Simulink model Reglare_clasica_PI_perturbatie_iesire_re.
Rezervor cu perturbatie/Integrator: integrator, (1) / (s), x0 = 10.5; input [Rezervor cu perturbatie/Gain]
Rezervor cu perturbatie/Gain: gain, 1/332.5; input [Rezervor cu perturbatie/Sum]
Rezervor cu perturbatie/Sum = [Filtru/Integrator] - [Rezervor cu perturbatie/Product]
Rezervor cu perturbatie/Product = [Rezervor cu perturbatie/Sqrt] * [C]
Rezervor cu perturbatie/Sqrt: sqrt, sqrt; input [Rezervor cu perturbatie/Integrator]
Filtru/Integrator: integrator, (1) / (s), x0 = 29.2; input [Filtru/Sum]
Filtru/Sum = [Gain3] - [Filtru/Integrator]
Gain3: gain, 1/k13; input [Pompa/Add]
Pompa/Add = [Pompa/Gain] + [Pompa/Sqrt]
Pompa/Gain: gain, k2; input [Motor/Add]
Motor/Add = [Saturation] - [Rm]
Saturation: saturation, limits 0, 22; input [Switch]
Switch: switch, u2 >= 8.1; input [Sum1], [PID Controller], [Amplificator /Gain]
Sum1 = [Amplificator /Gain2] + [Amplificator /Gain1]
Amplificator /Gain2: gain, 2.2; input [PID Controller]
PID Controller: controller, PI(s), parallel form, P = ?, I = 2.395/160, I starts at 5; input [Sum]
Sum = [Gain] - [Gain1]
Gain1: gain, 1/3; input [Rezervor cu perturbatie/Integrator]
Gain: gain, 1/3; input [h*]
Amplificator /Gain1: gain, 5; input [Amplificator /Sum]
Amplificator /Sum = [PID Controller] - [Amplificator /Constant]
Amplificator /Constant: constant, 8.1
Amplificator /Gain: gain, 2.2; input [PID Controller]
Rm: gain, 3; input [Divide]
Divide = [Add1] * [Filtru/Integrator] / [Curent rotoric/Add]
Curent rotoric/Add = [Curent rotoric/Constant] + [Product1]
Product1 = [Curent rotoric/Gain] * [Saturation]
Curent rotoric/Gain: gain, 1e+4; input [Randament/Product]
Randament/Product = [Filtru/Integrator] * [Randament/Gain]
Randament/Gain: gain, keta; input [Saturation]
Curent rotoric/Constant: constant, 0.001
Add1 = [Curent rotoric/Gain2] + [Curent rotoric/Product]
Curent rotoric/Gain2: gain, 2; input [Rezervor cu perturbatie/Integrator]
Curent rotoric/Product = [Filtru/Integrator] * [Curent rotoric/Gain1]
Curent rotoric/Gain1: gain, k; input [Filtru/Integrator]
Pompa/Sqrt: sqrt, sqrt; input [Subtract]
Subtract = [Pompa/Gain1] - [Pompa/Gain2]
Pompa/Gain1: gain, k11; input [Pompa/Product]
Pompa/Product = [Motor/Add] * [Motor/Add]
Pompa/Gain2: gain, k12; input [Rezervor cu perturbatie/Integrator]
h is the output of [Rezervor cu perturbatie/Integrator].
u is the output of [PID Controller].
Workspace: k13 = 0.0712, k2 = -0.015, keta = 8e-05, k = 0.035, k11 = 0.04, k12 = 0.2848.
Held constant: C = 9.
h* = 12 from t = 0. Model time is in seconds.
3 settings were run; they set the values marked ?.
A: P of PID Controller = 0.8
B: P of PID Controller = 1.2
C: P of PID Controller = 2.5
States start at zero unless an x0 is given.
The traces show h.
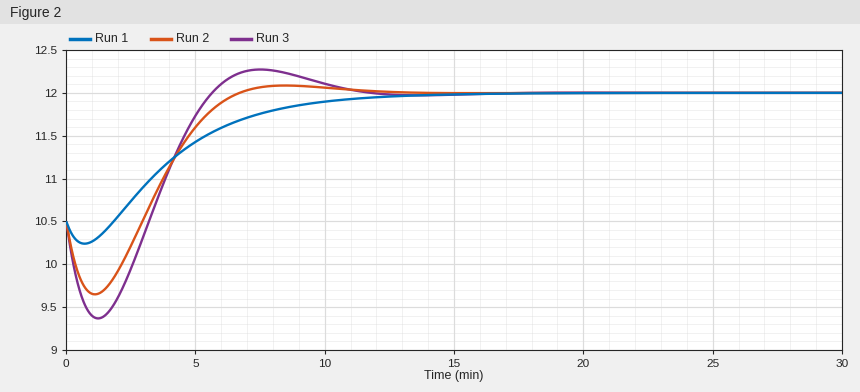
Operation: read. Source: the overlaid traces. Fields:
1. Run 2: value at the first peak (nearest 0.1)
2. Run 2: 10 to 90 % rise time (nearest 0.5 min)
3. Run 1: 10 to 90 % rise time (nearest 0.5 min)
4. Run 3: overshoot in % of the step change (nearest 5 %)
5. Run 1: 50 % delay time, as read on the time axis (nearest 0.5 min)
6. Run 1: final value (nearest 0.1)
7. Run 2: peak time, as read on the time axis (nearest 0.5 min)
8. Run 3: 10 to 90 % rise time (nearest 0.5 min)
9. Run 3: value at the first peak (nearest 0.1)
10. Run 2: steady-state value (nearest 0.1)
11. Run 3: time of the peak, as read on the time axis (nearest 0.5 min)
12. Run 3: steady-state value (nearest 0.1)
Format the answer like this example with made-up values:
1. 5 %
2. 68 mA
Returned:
1. 12.1
2. 2.5 min
3. 6.5 min
4. 20 %
5. 4.0 min
6. 12.0
7. 8.5 min
8. 2.0 min
9. 12.3
10. 12.0
11. 7.5 min
12. 12.0
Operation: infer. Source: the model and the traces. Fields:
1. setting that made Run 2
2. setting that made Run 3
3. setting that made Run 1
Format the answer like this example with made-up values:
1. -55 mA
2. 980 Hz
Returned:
1. B
2. A
3. C
